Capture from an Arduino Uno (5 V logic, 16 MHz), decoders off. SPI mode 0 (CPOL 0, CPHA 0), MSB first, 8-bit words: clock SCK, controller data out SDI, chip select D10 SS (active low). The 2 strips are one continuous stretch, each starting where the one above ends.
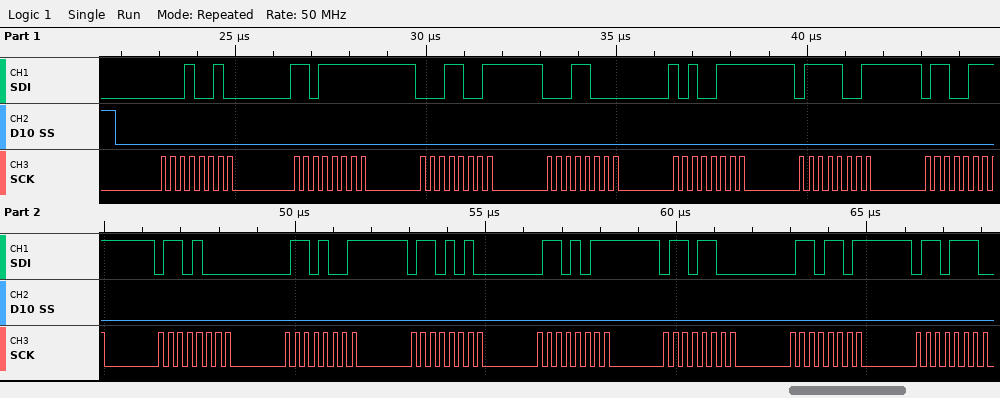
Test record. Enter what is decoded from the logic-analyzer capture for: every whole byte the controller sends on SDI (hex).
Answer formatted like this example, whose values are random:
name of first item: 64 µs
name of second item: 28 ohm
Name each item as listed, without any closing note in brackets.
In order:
every whole byte the controller sends on SDI: 0x12 0xDF 0x19 0x18 0xA7 0x79 0x67 0x68 0x69 0x6A 0x6B 0x6C 0x6D 0x6E
